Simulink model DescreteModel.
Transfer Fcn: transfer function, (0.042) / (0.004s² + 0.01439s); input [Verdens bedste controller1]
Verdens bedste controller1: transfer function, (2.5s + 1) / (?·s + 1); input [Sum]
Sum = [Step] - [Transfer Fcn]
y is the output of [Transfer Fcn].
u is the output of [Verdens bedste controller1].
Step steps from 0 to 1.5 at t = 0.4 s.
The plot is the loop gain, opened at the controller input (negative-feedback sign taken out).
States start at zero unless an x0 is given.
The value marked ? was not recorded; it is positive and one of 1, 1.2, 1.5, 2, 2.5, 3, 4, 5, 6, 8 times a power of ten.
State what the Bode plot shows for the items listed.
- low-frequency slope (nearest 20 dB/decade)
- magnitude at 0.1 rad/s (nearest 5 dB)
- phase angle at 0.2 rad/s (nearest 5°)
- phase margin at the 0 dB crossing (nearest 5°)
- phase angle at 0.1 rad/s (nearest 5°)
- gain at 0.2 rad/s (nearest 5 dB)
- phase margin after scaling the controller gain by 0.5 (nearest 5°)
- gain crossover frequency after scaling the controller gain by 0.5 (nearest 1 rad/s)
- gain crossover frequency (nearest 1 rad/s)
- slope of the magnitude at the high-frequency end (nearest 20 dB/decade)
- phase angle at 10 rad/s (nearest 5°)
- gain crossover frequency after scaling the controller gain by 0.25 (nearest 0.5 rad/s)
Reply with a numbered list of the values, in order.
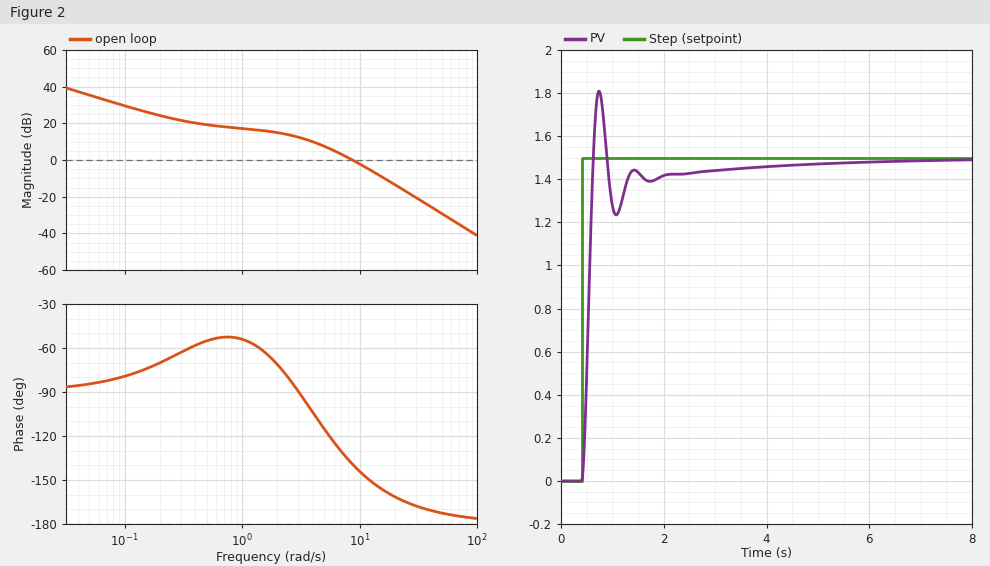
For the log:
1. -20 dB/decade
2. 30 dB
3. -70°
4. 40°
5. -80°
6. 25 dB
7. 60°
8. 6 rad/s
9. 9 rad/s
10. -40 dB/decade
11. -145°
12. 3.0 rad/s
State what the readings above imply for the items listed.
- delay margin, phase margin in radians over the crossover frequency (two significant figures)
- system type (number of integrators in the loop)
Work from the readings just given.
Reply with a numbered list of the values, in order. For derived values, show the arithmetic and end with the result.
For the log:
1. 40 × π / 180 / 9 = 0.078 s
2. 1
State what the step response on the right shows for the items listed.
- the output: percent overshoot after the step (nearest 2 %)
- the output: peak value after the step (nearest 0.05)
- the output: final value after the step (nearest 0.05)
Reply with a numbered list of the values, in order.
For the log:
1. 20 %
2. 1.80
3. 1.50
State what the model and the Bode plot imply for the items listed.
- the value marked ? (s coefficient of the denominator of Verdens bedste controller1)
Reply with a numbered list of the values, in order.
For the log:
1. 0.3
